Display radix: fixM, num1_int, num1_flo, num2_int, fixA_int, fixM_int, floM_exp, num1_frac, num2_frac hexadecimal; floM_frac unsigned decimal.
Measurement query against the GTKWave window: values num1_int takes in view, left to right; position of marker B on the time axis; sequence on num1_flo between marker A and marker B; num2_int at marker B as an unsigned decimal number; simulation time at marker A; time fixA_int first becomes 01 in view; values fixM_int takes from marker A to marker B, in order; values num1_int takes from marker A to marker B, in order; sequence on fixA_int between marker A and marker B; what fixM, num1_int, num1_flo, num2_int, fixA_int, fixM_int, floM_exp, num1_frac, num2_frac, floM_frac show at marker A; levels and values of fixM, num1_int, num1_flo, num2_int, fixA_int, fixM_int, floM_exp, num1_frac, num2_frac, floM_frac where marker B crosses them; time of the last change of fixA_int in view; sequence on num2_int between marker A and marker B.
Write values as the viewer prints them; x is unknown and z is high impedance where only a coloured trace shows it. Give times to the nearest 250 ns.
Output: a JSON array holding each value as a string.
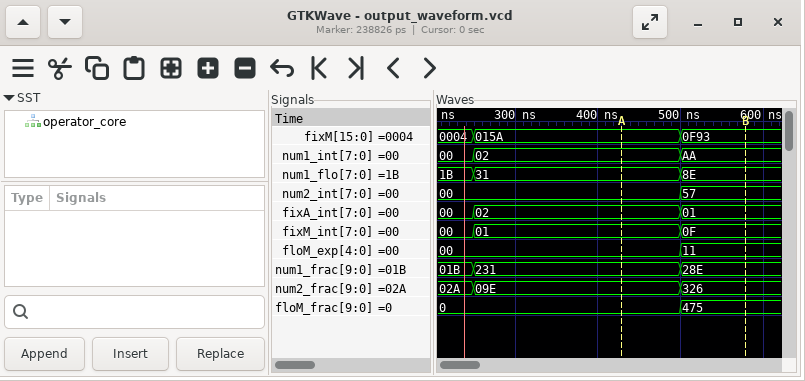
["00, 02, AA", "500 ns", "31, 8E", "87", "500 ns", "500 ns", "01, 0F", "02, AA", "02, 01", "fixM=015A, num1_int=02, num1_flo=31, num2_int=00, fixA_int=02, fixM_int=01, floM_exp=00, num1_frac=231, num2_frac=09E, floM_frac=0", "fixM=0F93, num1_int=AA, num1_flo=8E, num2_int=57, fixA_int=01, fixM_int=0F, floM_exp=11, num1_frac=28E, num2_frac=326, floM_frac=475", "500 ns", "00, 57"]
